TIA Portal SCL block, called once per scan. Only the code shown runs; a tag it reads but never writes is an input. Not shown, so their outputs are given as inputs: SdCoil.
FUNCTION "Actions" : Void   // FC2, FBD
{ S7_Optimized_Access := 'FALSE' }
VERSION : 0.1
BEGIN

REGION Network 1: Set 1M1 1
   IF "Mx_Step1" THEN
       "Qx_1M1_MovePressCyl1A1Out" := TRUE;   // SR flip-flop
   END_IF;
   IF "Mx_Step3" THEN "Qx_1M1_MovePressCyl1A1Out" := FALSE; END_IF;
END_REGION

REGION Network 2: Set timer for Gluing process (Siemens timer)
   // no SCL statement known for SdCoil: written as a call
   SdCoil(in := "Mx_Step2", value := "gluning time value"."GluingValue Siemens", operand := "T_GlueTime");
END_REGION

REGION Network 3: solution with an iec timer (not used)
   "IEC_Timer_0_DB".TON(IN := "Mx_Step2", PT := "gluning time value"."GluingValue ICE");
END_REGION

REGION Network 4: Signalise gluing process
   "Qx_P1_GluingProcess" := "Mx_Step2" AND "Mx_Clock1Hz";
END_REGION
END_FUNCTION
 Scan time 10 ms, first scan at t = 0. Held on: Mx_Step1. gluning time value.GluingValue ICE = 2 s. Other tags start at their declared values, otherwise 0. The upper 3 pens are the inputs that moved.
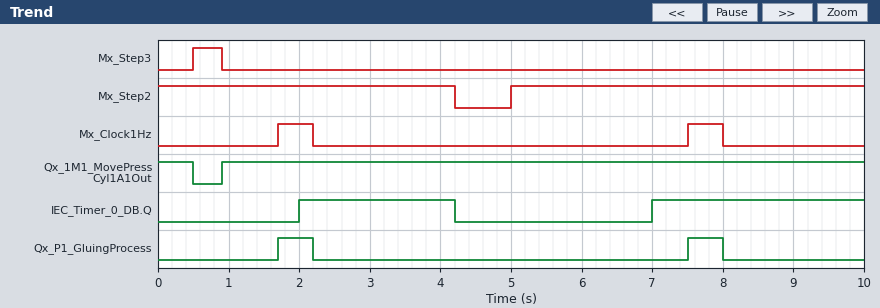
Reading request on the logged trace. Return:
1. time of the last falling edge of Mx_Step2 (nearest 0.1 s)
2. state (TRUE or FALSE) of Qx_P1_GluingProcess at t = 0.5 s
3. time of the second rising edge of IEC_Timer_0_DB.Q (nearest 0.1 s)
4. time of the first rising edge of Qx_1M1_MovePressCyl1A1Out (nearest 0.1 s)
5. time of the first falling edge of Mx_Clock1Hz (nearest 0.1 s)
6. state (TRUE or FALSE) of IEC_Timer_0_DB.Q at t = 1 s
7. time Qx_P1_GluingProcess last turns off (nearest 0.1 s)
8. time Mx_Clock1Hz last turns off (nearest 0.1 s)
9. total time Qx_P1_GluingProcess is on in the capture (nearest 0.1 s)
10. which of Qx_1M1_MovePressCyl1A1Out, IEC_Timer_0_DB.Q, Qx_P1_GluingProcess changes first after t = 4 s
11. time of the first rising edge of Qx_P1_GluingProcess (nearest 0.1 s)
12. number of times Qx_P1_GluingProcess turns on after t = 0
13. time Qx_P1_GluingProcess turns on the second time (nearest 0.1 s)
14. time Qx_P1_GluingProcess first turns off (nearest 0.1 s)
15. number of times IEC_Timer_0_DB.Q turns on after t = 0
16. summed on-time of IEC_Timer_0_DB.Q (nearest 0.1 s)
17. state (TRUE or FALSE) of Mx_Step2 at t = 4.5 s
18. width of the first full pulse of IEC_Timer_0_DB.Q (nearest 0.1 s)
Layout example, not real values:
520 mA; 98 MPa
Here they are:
4.2 s; FALSE; 7.0 s; 0.9 s; 2.2 s; FALSE; 8.0 s; 8.0 s; 1.0 s; IEC_Timer_0_DB.Q; 1.7 s; 2; 7.5 s; 2.2 s; 2; 5.2 s; FALSE; 2.2 s
